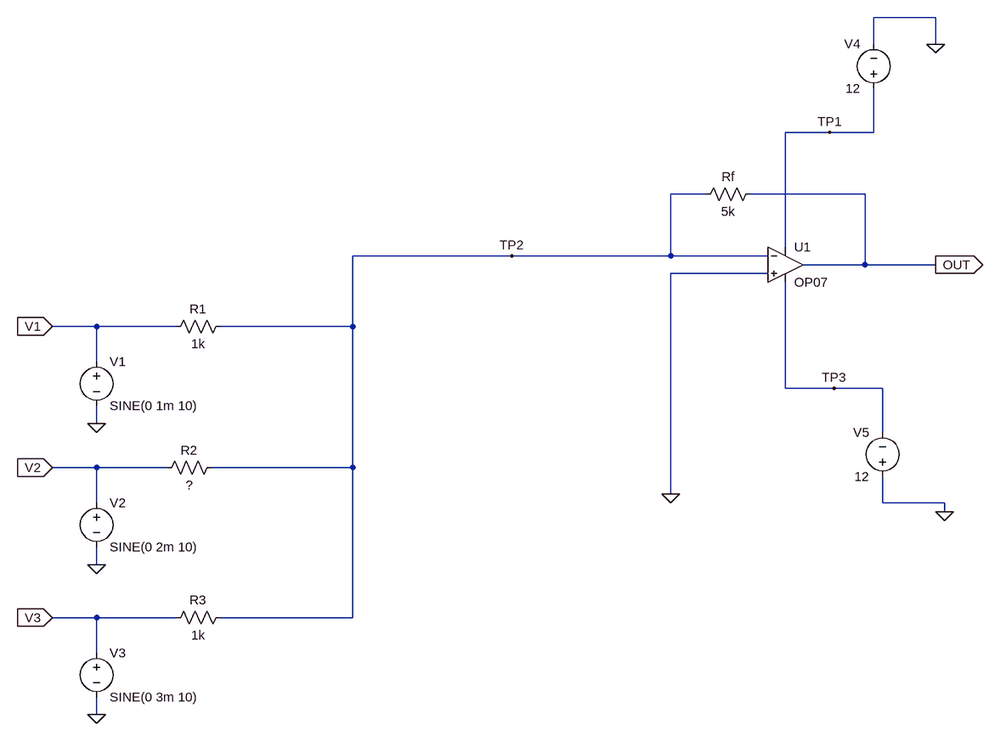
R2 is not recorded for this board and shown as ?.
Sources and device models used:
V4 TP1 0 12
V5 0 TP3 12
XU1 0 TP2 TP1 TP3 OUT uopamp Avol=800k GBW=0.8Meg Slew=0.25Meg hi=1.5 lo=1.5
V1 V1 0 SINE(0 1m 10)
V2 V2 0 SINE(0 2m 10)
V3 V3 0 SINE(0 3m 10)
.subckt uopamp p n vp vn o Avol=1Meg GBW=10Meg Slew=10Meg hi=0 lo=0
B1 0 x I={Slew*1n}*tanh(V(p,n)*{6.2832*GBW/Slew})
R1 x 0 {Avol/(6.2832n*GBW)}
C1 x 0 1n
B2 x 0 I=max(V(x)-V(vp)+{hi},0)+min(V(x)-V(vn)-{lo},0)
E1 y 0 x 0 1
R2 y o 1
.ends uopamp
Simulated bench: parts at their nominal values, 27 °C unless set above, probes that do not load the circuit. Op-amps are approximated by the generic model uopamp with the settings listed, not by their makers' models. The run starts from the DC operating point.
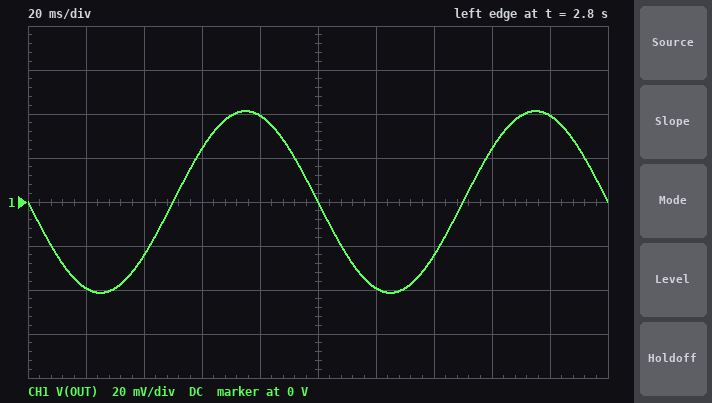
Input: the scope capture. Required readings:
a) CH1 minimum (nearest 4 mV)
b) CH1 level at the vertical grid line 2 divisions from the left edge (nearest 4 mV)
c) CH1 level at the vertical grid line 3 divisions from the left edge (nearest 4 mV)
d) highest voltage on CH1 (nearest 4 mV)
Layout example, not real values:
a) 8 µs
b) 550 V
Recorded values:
a) -40 mV
b) -24 mV
c) 24 mV
d) 40 mV
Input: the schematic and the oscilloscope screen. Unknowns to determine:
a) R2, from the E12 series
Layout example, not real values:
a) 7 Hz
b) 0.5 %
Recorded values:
a) 470 Ω
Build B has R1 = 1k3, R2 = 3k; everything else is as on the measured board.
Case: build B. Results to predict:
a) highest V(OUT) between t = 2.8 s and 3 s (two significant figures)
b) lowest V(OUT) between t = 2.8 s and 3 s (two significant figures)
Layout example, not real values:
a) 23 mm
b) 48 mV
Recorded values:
a) 22 mV
b) -22 mV
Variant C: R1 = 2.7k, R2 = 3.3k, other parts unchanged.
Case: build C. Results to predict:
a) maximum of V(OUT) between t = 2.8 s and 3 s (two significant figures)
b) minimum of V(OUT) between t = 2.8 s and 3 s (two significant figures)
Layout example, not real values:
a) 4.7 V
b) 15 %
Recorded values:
a) 20 mV
b) -20 mV
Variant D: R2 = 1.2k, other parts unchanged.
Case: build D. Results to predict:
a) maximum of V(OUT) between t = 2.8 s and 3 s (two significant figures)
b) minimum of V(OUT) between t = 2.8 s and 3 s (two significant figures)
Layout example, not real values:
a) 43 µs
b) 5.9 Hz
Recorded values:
a) 28 mV
b) -28 mV
